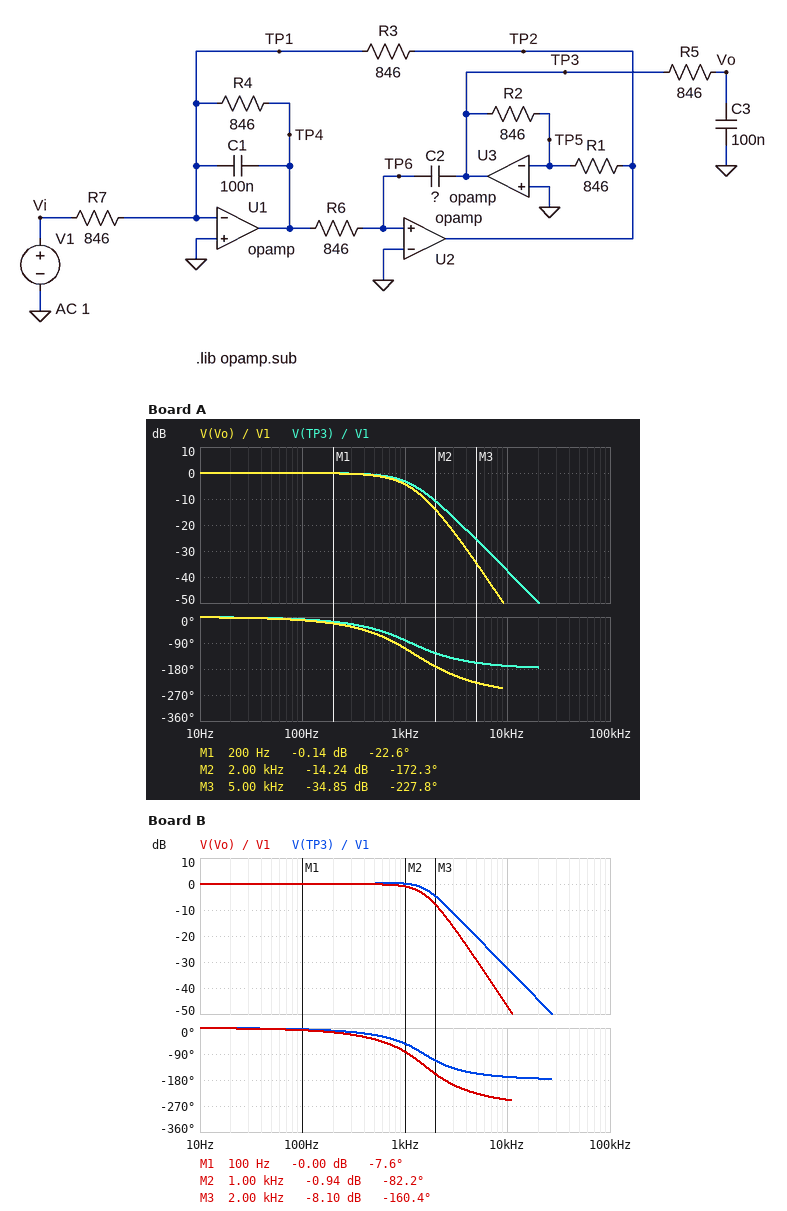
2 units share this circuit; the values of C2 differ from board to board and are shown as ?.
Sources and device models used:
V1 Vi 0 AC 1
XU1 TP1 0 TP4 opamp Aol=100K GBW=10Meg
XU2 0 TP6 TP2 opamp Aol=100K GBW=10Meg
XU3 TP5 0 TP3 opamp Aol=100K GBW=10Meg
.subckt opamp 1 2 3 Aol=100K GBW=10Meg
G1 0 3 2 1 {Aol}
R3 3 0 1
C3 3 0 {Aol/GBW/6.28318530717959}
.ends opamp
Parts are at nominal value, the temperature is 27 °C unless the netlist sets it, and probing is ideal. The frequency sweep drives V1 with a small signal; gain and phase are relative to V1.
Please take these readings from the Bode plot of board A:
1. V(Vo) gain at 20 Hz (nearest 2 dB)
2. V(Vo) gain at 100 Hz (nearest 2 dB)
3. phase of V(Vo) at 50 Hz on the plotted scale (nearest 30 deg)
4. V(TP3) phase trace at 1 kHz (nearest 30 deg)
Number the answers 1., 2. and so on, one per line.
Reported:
1. 0 dB
2. 0 dB
3. 0 deg
4. -90 deg
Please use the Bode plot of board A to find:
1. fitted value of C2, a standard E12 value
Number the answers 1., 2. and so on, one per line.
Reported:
1. 270 nF
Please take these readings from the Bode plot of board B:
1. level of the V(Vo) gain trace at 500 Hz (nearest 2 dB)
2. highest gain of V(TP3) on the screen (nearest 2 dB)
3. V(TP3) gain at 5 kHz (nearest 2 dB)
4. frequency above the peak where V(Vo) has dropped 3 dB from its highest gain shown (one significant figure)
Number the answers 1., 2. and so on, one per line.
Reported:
1. 0 dB
2. 0 dB
3. -20 dB
4. 1 kHz
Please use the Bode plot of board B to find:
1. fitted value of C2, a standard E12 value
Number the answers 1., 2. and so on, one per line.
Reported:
1. 150 nF
